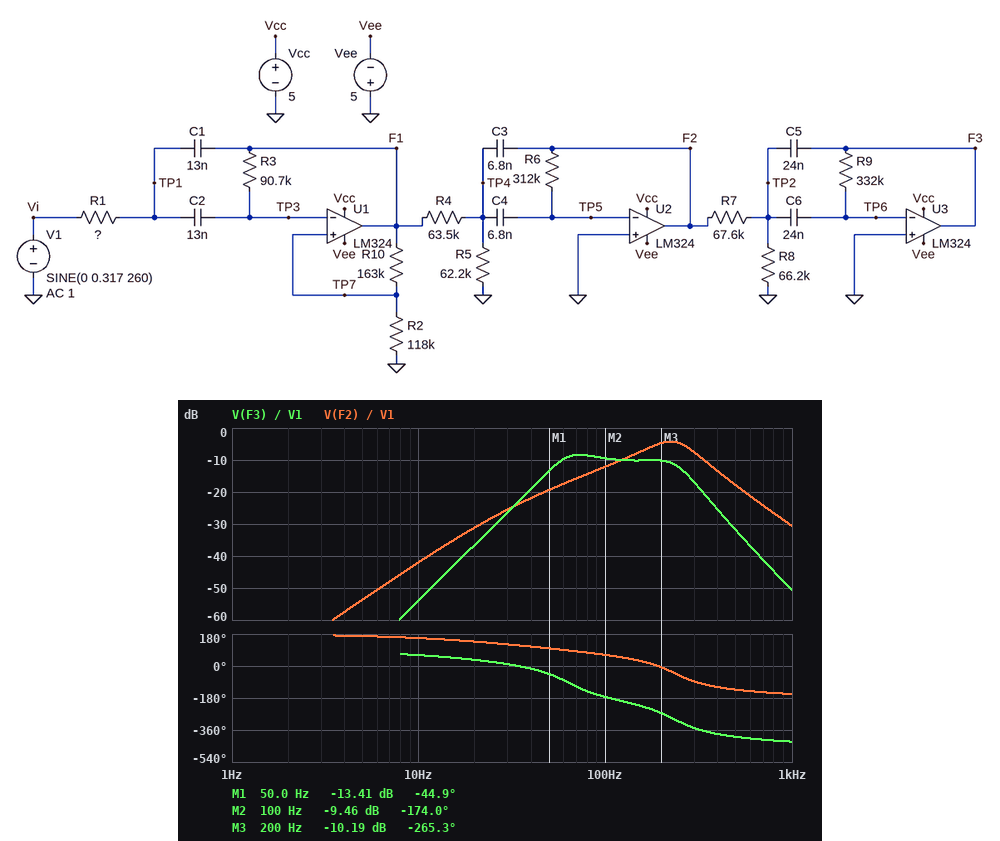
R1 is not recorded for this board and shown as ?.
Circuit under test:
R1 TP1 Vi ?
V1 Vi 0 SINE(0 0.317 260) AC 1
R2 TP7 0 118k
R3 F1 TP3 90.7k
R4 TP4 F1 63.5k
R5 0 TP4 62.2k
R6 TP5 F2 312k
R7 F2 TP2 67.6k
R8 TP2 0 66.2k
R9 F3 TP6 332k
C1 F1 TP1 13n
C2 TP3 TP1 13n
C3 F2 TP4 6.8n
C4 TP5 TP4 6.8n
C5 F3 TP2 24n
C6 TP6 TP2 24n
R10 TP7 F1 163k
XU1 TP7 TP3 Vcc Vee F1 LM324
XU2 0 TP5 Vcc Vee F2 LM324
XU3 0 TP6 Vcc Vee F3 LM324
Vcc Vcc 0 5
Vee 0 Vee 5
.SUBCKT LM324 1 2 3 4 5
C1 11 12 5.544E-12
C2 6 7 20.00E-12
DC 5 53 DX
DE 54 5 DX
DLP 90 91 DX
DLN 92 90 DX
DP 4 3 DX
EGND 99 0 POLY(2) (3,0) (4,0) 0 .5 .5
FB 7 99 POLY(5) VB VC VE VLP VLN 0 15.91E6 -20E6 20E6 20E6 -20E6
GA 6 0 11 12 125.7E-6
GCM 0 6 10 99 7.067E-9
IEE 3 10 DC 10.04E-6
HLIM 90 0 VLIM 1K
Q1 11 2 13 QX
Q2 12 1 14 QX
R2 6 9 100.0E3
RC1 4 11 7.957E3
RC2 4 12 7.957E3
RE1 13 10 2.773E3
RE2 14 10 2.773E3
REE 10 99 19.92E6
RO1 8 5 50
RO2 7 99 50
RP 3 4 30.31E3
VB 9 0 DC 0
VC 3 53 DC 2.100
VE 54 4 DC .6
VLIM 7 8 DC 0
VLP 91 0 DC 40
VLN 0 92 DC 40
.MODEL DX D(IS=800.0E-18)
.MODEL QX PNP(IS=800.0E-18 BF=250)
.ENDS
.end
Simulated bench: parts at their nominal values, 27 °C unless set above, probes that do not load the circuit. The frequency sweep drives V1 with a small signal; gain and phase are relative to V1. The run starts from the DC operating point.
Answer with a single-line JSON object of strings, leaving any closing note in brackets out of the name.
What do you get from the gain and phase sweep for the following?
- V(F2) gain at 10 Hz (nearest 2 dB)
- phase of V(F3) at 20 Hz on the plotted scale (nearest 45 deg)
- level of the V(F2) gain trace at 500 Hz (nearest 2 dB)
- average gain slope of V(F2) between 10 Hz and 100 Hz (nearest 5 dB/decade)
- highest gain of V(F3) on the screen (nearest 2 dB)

{"V(F2) gain at 10 Hz": "-42 dB", "phase of V(F3) at 20 Hz on the plotted scale": "45 deg", "level of the V(F2) gain trace at 500 Hz": "-18 dB", "average gain slope of V(F2) between 10 Hz and 100 Hz": "30 dB/decade", "highest gain of V(F3) on the screen": "-8 dB"}
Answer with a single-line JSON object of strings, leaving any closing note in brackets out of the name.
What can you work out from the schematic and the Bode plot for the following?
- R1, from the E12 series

{"R1, from the E12 series": "270 kΩ"}
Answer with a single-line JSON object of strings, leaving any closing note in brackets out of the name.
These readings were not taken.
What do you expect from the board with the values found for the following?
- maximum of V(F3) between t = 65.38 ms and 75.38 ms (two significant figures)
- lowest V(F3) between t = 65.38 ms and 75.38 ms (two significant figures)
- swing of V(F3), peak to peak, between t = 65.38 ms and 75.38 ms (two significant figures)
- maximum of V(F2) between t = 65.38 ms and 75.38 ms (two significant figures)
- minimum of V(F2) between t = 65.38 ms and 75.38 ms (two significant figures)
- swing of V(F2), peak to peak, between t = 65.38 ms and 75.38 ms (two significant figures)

{"maximum of V(F3) between t = 65.38 ms and 75.38 ms": "62 mV", "lowest V(F3) between t = 65.38 ms and 75.38 ms": "-75 mV", "swing of V(F3), peak to peak, between t = 65.38 ms and 75.38 ms": "140 mV", "maximum of V(F2) between t = 65.38 ms and 75.38 ms": "170 mV", "minimum of V(F2) between t = 65.38 ms and 75.38 ms": "-180 mV", "swing of V(F2), peak to peak, between t = 65.38 ms and 75.38 ms": "350 mV"}
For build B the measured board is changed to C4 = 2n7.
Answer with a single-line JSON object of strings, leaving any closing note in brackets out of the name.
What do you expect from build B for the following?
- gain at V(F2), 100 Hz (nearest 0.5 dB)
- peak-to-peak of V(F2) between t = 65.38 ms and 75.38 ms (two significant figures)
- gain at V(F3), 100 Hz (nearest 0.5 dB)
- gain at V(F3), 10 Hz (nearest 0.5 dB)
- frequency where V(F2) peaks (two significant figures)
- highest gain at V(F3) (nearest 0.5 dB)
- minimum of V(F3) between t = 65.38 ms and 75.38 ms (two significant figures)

{"gain at V(F2), 100 Hz": "-21.0 dB", "peak-to-peak of V(F2) between t = 65.38 ms and 75.38 ms": "140 mV", "gain at V(F3), 100 Hz": "-18.5 dB", "gain at V(F3), 10 Hz": "-62.0 dB", "frequency where V(F2) peaks": "340 Hz", "highest gain at V(F3)": "-17.0 dB", "minimum of V(F3) between t = 65.38 ms and 75.38 ms": "-35 mV"}
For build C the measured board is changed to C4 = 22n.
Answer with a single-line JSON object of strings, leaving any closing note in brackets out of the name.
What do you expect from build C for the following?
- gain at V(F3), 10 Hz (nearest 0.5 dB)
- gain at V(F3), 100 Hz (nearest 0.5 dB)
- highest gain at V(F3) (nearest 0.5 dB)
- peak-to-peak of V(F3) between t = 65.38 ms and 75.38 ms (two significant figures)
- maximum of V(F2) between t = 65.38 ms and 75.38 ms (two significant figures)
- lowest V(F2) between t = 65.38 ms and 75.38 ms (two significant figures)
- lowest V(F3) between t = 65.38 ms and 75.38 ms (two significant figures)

{"gain at V(F3), 10 Hz": "-43.5 dB", "gain at V(F3), 100 Hz": "2.5 dB", "highest gain at V(F3)": "3.0 dB", "peak-to-peak of V(F3) between t = 65.38 ms and 75.38 ms": "99 mV", "maximum of V(F2) between t = 65.38 ms and 75.38 ms": "120 mV", "lowest V(F2) between t = 65.38 ms and 75.38 ms": "-130 mV", "lowest V(F3) between t = 65.38 ms and 75.38 ms": "-56 mV"}
